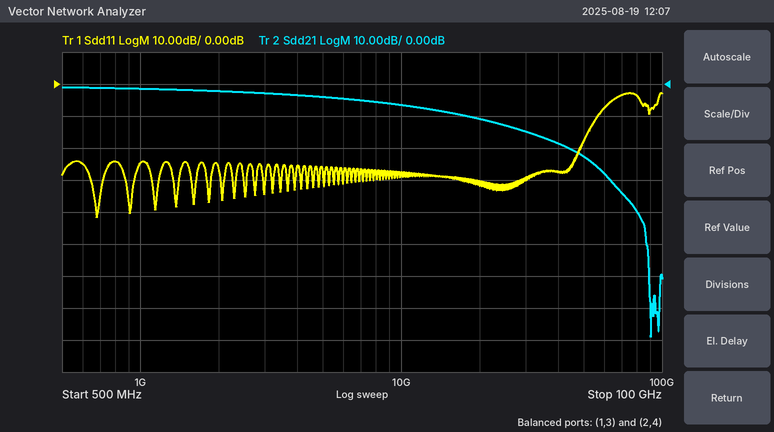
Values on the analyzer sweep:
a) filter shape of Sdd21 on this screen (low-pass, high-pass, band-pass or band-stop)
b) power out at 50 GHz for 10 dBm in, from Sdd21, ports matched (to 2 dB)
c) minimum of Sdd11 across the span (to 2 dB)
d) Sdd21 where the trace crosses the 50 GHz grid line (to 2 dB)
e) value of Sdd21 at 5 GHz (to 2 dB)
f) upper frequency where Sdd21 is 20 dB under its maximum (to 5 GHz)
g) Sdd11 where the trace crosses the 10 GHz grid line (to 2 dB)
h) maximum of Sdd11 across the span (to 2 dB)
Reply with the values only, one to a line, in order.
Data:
low-pass
-12 dBm
-42 dB
-22 dB
-4 dB
45 GHz
-28 dB
-2 dB
